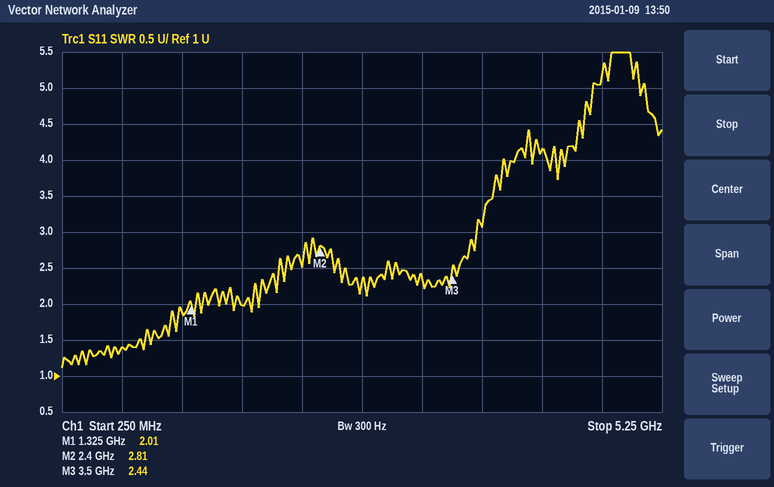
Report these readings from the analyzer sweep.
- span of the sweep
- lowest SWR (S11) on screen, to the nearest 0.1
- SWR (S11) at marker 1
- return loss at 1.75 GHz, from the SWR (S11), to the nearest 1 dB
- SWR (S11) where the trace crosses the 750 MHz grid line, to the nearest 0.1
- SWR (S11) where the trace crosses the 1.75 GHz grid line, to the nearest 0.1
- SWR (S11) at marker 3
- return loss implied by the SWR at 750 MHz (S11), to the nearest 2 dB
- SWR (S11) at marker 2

5 GHz
1.1
2.01
10 dB
1.4
2.0
2.44
16 dB
2.81
